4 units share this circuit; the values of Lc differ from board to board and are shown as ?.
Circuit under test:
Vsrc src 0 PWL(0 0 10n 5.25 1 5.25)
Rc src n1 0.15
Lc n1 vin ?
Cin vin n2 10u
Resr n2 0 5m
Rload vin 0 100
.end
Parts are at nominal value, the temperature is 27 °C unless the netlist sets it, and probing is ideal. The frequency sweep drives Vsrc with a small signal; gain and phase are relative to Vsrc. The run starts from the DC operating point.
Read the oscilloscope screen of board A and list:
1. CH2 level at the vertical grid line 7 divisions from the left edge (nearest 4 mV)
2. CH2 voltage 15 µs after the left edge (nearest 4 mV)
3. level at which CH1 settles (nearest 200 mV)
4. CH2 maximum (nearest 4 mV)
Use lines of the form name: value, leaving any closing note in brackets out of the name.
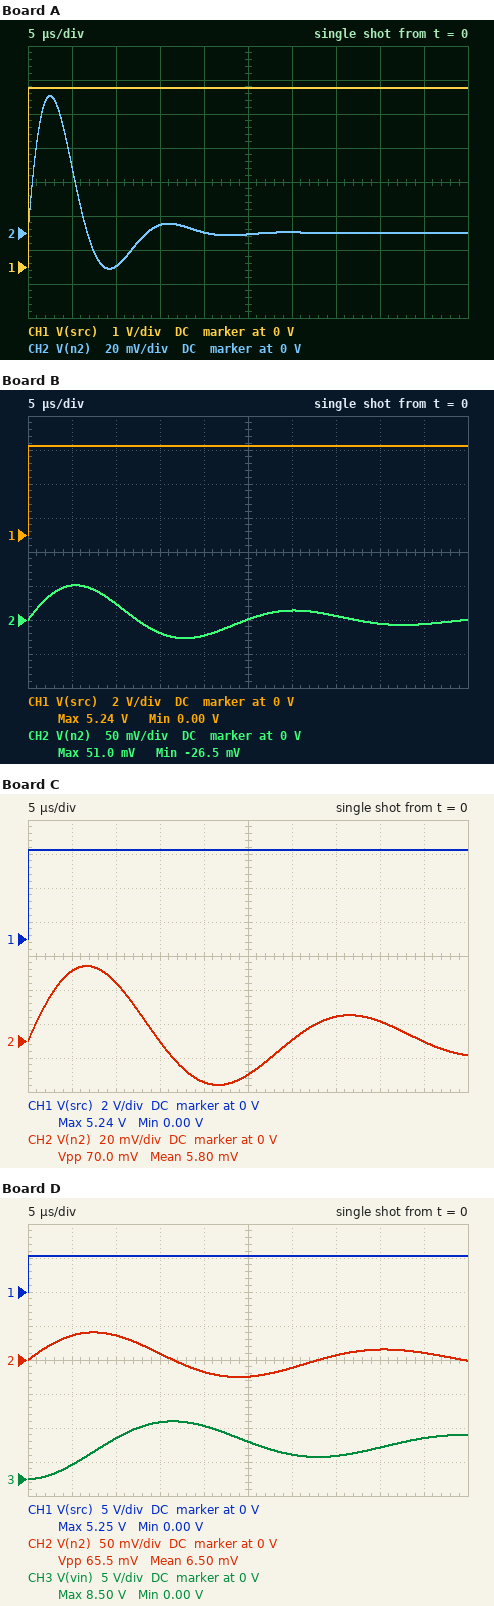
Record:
CH2 level at the vertical grid line 7 divisions from the left edge: 0 V
CH2 voltage 15 µs after the left edge: 4 mV
level at which CH1 settles: 5.2 V
CH2 maximum: 80 mV
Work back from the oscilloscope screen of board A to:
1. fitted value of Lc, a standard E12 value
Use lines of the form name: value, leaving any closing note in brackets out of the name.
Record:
fitted value of Lc, a standard E12 value: 390 nH
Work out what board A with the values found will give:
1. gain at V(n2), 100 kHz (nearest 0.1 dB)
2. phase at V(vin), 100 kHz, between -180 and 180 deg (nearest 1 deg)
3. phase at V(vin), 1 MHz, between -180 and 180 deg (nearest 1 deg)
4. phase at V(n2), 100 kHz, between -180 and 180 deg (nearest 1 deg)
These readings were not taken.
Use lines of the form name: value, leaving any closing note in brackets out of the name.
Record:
gain at V(n2), 100 kHz: -31.0 dB
phase at V(vin), 100 kHz, between -180 and 180 deg: -117 deg
phase at V(vin), 1 MHz, between -180 and 180 deg: -159 deg
phase at V(n2), 100 kHz, between -180 and 180 deg: -29 deg
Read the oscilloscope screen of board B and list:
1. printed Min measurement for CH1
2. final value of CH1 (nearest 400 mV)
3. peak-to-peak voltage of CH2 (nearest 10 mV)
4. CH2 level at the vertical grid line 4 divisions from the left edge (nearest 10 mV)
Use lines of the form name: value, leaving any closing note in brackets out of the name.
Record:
printed Min measurement for CH1: 0.00 V
final value of CH1: 5.2 V
peak-to-peak voltage of CH2: 80 mV
CH2 level at the vertical grid line 4 divisions from the left edge: -20 mV
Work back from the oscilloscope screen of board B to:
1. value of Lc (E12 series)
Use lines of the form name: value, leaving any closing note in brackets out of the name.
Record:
value of Lc: 1.5 µH
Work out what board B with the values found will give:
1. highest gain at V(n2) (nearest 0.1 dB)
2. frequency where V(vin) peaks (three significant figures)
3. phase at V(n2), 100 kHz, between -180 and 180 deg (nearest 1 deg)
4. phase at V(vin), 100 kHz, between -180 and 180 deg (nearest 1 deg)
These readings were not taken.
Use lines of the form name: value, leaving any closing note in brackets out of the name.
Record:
highest gain at V(n2): -29.9 dB
frequency where V(vin) peaks: 39.4 kHz
phase at V(n2), 100 kHz, between -180 and 180 deg: -79 deg
phase at V(vin), 100 kHz, between -180 and 180 deg: -167 deg
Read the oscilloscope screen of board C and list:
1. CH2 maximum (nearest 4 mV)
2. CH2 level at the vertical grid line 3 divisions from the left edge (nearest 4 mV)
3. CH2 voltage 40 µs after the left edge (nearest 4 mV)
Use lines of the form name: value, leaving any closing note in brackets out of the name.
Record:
CH2 maximum: 44 mV
CH2 level at the vertical grid line 3 divisions from the left edge: 0 V
CH2 voltage 40 µs after the left edge: 12 mV
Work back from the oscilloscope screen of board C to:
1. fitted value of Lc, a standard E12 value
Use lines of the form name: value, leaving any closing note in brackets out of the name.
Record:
fitted value of Lc, a standard E12 value: 2.2 µH
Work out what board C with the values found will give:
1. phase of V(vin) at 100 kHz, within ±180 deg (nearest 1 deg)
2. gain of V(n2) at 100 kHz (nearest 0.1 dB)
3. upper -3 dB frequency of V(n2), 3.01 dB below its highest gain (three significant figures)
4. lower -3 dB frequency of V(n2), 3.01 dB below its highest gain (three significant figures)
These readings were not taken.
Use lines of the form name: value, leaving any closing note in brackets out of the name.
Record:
phase of V(vin) at 100 kHz, within ±180 deg: -171 deg
gain of V(n2) at 100 kHz: -47.8 dB
upper -3 dB frequency of V(n2), 3.01 dB below its highest gain: 40.1 kHz
lower -3 dB frequency of V(n2), 3.01 dB below its highest gain: 28.7 kHz
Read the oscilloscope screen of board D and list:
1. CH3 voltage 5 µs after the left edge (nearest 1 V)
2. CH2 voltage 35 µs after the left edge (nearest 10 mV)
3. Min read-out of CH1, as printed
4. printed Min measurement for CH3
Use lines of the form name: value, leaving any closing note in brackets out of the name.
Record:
CH3 voltage 5 µs after the left edge: 2 V
CH2 voltage 35 µs after the left edge: 10 mV
Min read-out of CH1, as printed: 0.00 V
printed Min measurement for CH3: 0.00 V
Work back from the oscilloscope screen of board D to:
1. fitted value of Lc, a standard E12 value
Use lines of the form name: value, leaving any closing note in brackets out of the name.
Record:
fitted value of Lc, a standard E12 value: 2.7 µH
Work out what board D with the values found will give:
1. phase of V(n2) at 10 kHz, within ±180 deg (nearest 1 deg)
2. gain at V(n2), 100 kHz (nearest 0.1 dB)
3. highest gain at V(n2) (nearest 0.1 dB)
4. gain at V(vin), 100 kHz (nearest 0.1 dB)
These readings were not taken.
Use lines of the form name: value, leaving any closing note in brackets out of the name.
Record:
phase of V(n2) at 10 kHz, within ±180 deg: 84 deg
gain at V(n2), 100 kHz: -49.8 dB
highest gain at V(n2): -30.0 dB
gain at V(vin), 100 kHz: -19.7 dB
